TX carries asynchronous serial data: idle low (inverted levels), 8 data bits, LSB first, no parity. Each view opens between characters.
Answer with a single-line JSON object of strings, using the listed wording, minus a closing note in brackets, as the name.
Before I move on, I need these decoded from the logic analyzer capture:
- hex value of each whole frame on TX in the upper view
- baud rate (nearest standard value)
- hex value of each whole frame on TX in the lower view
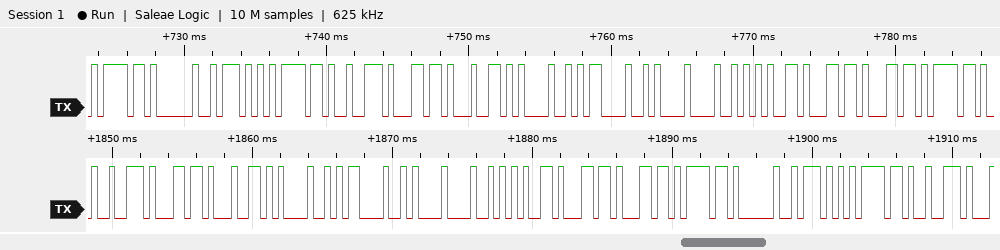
{"hex value of each whole frame on TX in the upper view": "21, BF, 51, 21, 1B, 27, 37, BD, E5, EB, 6F, 35, 27, 27, 21", "baud rate": "2400 baud", "hex value of each whole frame on TX in the lower view": "1B, 27, 37, BD, E5, EB, 6F, 35, 27, 27, 21, BF, 51, 21, 1B"}
